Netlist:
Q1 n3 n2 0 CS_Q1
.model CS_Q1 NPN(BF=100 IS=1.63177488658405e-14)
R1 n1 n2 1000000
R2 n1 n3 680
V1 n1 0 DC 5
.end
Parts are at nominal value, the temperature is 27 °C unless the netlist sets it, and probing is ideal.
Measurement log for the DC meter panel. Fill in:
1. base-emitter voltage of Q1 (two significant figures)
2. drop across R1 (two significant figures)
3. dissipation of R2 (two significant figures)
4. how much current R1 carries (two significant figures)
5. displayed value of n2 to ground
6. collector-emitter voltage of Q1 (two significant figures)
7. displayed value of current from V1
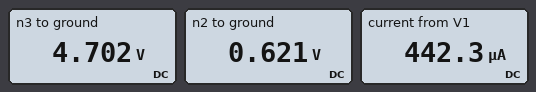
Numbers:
620 mV
4.4 V
130 µW
4.4 µA
0.621 V
4.7 V
442.3 µA
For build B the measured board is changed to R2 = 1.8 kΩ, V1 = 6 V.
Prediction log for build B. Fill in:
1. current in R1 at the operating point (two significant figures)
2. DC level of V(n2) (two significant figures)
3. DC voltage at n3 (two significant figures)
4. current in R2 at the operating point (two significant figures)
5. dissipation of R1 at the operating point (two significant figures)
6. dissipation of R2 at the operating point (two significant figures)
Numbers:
5.4 µA
630 mV
5.0 V
540 µA
29 µW
520 µW
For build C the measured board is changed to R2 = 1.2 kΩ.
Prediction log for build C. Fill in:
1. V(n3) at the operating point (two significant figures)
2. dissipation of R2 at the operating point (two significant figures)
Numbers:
4.5 V
230 µW
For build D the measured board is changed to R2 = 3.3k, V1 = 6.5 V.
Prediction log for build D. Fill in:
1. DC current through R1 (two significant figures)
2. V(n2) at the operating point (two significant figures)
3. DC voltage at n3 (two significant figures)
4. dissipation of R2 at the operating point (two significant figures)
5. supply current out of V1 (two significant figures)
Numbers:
5.9 µA
630 mV
4.6 V
1.1 mW
590 µA
